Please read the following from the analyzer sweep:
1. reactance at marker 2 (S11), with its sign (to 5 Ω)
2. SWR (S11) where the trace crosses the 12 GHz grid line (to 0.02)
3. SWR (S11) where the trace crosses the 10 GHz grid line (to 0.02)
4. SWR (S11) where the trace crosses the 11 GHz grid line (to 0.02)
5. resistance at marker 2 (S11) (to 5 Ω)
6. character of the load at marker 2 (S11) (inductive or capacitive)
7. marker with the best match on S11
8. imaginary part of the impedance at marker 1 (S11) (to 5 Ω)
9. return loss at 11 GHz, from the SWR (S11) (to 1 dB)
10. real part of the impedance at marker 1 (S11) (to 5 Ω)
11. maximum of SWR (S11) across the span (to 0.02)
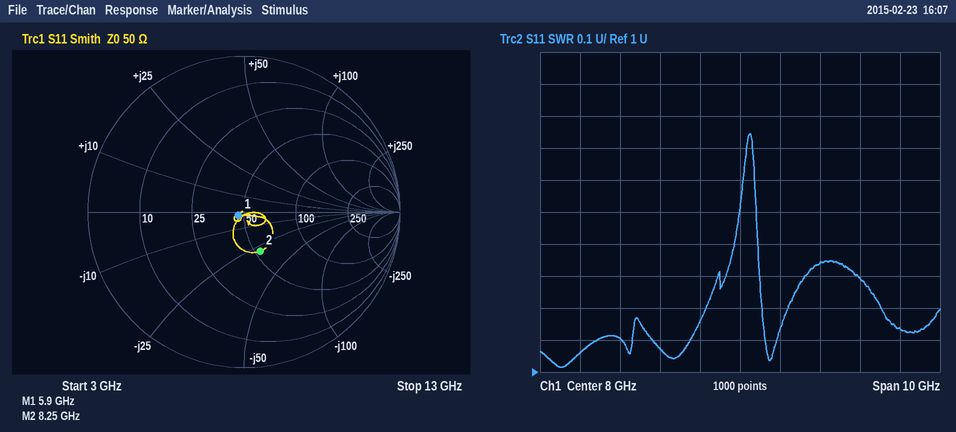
-30 Ω
1.14
1.34
1.30
55 Ω
capacitive
marker 1
0 Ω
18 dB
45 Ω
1.74
